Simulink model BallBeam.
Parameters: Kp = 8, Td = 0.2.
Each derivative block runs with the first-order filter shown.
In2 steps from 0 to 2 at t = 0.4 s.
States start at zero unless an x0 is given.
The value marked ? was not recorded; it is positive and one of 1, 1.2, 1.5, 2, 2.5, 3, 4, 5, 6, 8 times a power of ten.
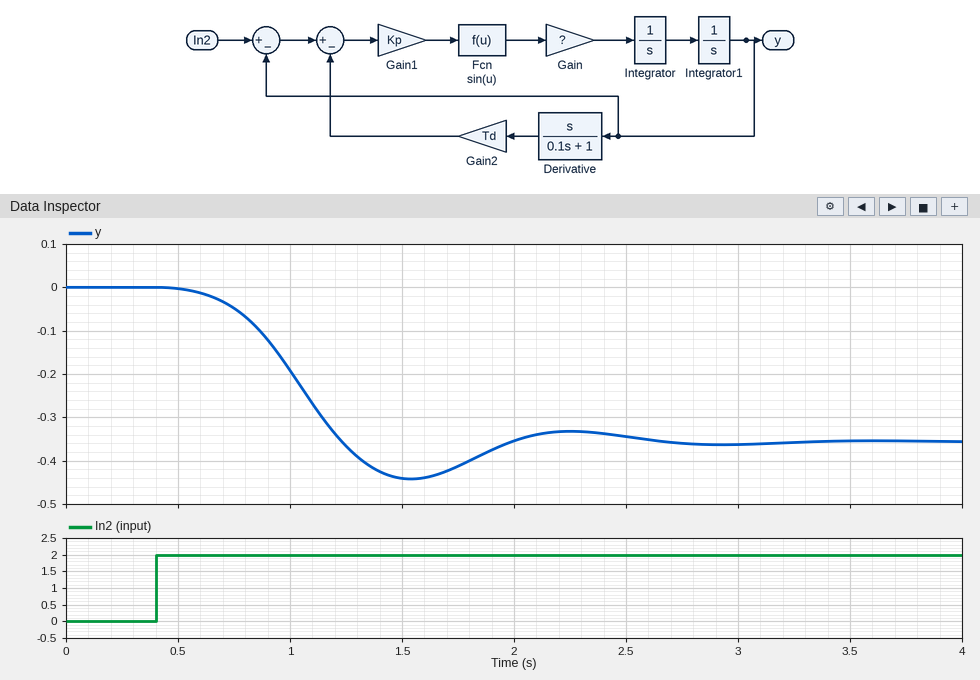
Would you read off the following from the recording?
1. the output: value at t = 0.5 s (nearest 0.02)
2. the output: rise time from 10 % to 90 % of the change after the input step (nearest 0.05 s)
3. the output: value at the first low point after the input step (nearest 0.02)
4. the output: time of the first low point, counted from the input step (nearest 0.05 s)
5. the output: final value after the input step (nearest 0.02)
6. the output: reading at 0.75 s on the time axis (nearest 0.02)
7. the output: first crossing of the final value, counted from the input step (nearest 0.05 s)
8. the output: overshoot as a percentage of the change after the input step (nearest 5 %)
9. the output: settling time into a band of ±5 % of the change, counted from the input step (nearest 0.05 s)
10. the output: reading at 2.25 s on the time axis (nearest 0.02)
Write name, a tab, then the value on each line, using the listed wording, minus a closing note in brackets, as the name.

the output: value at t = 0.5 s	0.00
the output: rise time from 10 % to 90 % of the change after the input step	0.45 s
the output: value at the first low point after the input step	-0.44
the output: time of the first low point, counted from the input step	1.15 s
the output: final value after the input step	-0.36
the output: reading at 0.75 s on the time axis	-0.04
the output: first crossing of the final value, counted from the input step	0.85 s
the output: overshoot as a percentage of the change after the input step	25 %
the output: settling time into a band of ±5 % of the change, counted from the input step	2.00 s
the output: reading at 2.25 s on the time axis	-0.34
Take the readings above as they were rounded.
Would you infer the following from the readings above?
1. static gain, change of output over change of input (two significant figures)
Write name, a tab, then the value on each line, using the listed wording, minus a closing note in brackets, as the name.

static gain, change of output over change of input	-0.18
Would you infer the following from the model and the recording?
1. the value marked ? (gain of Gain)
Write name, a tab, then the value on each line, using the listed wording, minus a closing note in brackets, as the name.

the value marked ?	2
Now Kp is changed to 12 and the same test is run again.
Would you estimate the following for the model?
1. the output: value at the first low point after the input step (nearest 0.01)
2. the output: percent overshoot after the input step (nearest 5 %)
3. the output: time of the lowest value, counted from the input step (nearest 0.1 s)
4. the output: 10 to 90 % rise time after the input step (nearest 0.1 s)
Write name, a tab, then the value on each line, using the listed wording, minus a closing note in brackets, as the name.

the output: value at the first low point after the input step	-0.11
the output: percent overshoot after the input step	15 %
the output: time of the lowest value, counted from the input step	0.6 s
the output: 10 to 90 % rise time after the input step	0.3 s
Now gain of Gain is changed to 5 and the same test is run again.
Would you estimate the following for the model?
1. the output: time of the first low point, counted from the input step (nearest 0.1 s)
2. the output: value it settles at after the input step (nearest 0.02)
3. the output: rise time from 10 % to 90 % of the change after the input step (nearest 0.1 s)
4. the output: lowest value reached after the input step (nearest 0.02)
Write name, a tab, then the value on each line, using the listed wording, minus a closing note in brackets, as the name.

the output: time of the first low point, counted from the input step	0.7 s
the output: value it settles at after the input step	-0.36
the output: rise time from 10 % to 90 % of the change after the input step	0.3 s
the output: lowest value reached after the input step	-0.38
